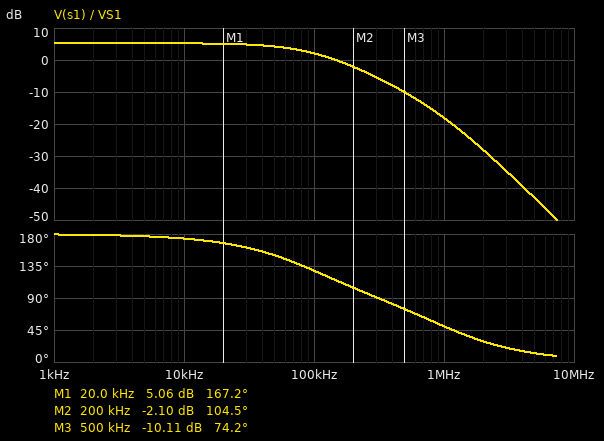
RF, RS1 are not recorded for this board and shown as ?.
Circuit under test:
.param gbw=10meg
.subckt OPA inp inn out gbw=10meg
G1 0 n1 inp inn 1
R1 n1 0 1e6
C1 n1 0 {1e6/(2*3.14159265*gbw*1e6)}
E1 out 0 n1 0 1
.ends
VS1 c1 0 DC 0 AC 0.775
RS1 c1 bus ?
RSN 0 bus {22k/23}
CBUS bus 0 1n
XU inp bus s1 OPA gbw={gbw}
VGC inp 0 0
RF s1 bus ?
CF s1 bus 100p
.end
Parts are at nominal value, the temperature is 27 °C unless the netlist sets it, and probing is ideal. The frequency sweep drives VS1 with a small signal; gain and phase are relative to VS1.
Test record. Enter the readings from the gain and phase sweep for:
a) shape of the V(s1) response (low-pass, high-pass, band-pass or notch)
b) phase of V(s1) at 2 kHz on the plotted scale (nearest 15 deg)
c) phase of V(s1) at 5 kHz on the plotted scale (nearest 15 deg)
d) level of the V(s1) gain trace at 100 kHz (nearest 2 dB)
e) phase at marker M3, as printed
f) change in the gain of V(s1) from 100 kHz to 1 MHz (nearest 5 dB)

low-pass
180 deg
180 deg
2 dB
74.2 deg
-20 dB
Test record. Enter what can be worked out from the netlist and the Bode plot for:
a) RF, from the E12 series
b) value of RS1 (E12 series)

15 kΩ
8.2 kΩ
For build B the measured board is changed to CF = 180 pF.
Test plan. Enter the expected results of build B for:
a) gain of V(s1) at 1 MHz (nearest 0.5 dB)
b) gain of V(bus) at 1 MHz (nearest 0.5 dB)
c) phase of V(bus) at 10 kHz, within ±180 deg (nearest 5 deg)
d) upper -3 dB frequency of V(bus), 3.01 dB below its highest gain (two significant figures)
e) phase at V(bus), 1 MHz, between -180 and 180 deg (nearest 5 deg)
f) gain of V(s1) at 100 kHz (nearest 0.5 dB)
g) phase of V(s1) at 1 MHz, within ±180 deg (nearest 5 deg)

-21.5 dB
-41.5 dB
80 deg
1.7 MHz
-30 deg
-1.0 dB
60 deg
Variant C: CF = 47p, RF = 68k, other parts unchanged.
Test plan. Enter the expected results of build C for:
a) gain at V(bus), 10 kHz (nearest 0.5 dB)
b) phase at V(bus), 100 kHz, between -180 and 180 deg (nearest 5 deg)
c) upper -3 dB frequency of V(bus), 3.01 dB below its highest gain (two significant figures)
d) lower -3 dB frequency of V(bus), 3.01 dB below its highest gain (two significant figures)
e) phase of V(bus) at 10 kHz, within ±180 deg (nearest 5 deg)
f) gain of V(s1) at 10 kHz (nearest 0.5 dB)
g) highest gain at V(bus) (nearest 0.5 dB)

-42.0 dB
10 deg
660 kHz
34 kHz
75 deg
18.0 dB
-30.5 dB
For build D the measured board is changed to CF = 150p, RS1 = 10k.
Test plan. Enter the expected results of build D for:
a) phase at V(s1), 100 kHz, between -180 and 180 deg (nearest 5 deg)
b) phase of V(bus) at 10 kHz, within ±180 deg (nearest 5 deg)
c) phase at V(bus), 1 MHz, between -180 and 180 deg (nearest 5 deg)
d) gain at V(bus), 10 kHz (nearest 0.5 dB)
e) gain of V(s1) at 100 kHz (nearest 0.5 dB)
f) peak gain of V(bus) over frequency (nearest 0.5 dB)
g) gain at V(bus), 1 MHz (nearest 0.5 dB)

120 deg
80 deg
-30 deg
-56.5 dB
-1.5 dB
-40.5 dB
-42.0 dB
